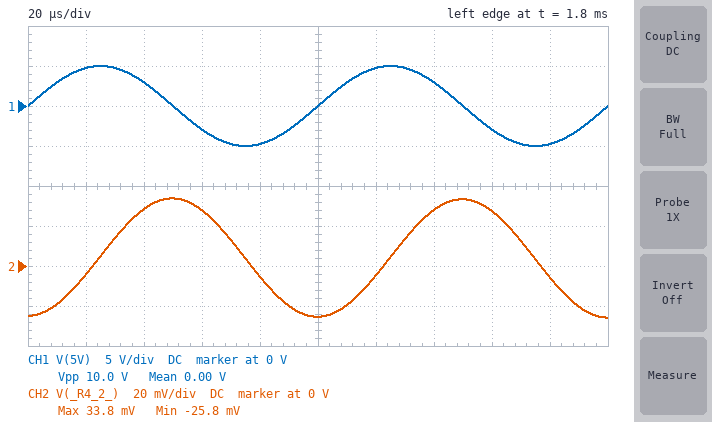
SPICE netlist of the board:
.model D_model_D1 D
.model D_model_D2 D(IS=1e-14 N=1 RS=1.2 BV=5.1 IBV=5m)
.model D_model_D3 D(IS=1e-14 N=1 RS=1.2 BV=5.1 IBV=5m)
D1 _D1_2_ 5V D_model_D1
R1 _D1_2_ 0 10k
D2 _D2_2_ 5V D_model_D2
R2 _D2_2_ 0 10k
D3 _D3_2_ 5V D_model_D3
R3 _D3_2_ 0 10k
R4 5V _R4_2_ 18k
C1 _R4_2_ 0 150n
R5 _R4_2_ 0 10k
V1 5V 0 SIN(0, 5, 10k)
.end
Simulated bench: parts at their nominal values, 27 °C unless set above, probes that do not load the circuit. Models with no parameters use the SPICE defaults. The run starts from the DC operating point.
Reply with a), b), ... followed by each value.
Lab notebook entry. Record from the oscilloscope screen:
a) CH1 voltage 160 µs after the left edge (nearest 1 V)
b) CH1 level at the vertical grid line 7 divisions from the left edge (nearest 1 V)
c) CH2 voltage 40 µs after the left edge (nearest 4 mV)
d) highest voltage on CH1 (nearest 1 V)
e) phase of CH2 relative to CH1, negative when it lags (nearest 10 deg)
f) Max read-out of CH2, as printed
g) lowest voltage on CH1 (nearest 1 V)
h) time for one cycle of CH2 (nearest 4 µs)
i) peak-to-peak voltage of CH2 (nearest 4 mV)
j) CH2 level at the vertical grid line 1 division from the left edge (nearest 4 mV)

a) -3 V
b) 3 V
c) 28 mV
d) 5 V
e) -90 deg
f) 33.8 mV
g) -5 V
h) 100 µs
i) 60 mV
j) -4 mV
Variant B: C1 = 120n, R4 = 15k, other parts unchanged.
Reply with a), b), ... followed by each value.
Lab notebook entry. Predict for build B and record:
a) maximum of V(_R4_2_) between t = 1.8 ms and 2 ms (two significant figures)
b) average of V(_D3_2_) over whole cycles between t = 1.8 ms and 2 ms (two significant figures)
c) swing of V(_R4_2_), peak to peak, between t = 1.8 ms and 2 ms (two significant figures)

a) 48 mV
b) -1.3 V
c) 89 mV
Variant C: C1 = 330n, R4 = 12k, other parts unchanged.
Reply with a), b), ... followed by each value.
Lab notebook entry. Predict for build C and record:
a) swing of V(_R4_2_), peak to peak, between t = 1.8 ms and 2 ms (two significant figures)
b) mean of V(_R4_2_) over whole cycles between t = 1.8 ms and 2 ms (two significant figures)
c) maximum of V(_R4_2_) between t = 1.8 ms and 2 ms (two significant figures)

a) 41 mV
b) 7.1 mV
c) 27 mV
